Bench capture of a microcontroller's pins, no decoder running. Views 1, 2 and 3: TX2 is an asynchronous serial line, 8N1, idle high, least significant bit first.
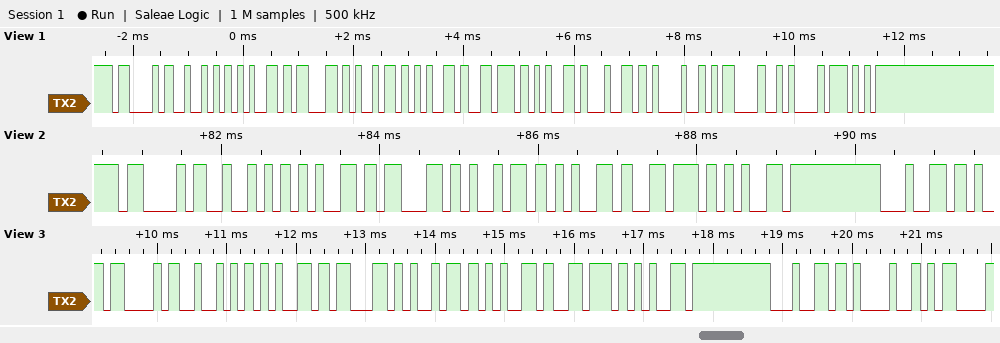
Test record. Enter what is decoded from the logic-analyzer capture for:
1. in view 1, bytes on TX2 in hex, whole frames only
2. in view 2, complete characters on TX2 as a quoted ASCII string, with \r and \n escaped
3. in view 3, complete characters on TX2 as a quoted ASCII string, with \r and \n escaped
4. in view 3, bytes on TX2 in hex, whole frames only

43 52 65 63 69 65 76 65 64 21 0D 0A 57
"CRecieved"
"CRecieved!\r"
43 52 65 63 69 65 76 65 64 21 0D
